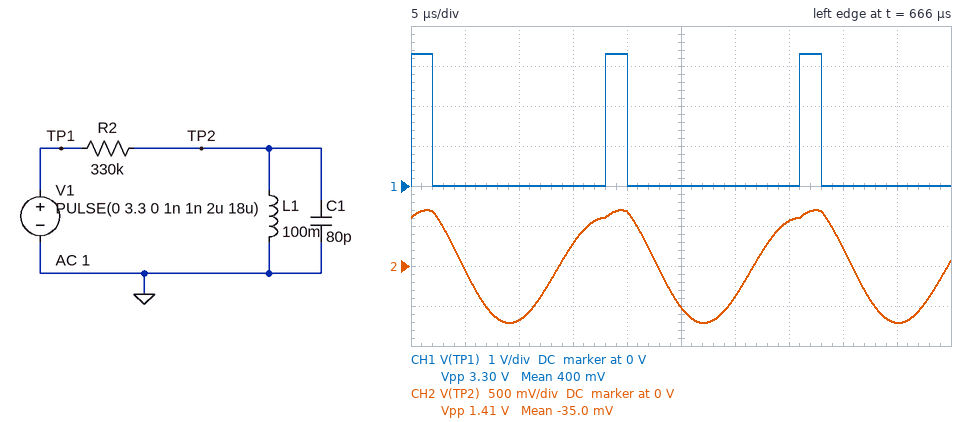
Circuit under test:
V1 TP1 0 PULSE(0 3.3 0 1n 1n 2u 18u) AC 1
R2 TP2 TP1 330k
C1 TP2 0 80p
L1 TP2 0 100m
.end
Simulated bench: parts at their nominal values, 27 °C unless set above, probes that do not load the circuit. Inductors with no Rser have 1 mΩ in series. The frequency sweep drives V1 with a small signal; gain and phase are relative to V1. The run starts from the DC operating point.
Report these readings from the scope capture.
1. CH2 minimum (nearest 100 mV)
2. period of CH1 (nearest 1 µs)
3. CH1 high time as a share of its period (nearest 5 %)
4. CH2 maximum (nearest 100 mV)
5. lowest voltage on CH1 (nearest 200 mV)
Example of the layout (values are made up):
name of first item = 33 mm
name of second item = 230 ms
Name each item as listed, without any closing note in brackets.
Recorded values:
CH2 minimum = -700 mV
period of CH1 = 18 µs
CH1 high time as a share of its period = 10 %
CH2 maximum = 700 mV
lowest voltage on CH1 = 0 V
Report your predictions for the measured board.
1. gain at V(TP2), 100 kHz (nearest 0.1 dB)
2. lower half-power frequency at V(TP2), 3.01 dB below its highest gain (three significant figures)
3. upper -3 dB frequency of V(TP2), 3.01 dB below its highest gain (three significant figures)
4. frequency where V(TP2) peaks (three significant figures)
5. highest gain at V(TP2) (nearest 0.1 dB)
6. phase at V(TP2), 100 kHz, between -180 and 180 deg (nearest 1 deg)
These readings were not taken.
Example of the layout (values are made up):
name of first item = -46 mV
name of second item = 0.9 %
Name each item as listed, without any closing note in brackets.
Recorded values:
gain at V(TP2), 100 kHz = -21.1 dB
lower half-power frequency at V(TP2), 3.01 dB below its highest gain = 53.3 kHz
upper -3 dB frequency of V(TP2), 3.01 dB below its highest gain = 59.4 kHz
frequency where V(TP2) peaks = 56.3 kHz
highest gain at V(TP2) = 0 dB
phase at V(TP2), 100 kHz, between -180 and 180 deg = -85 deg
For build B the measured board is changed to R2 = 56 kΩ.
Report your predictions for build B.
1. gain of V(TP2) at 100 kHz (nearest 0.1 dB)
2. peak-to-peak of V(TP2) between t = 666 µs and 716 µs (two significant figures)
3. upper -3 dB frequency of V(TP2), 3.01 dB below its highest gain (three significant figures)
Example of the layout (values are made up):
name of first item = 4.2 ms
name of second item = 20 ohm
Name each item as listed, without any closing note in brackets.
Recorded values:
gain of V(TP2) at 100 kHz = -6.7 dB
peak-to-peak of V(TP2) between t = 666 µs and 716 µs = 2.0 V
upper -3 dB frequency of V(TP2), 3.01 dB below its highest gain = 76.8 kHz
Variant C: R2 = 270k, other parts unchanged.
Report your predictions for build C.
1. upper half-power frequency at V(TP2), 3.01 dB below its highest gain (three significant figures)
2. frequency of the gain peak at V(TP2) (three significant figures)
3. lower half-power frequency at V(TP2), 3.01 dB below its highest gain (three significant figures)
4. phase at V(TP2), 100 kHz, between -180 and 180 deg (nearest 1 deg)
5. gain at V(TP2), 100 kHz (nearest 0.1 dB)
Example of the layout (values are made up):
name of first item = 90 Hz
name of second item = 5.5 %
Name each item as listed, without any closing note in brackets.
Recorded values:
upper half-power frequency at V(TP2), 3.01 dB below its highest gain = 60.1 kHz
frequency of the gain peak at V(TP2) = 56.3 kHz
lower half-power frequency at V(TP2), 3.01 dB below its highest gain = 52.7 kHz
phase at V(TP2), 100 kHz, between -180 and 180 deg = -84 deg
gain at V(TP2), 100 kHz = -19.4 dB
